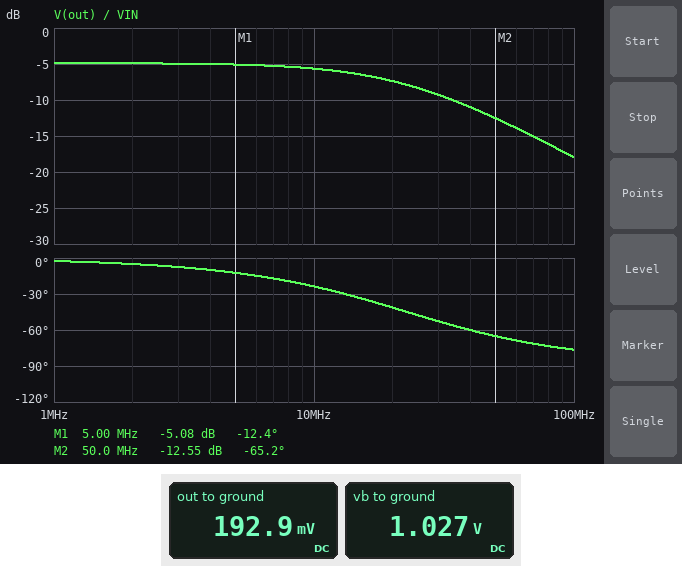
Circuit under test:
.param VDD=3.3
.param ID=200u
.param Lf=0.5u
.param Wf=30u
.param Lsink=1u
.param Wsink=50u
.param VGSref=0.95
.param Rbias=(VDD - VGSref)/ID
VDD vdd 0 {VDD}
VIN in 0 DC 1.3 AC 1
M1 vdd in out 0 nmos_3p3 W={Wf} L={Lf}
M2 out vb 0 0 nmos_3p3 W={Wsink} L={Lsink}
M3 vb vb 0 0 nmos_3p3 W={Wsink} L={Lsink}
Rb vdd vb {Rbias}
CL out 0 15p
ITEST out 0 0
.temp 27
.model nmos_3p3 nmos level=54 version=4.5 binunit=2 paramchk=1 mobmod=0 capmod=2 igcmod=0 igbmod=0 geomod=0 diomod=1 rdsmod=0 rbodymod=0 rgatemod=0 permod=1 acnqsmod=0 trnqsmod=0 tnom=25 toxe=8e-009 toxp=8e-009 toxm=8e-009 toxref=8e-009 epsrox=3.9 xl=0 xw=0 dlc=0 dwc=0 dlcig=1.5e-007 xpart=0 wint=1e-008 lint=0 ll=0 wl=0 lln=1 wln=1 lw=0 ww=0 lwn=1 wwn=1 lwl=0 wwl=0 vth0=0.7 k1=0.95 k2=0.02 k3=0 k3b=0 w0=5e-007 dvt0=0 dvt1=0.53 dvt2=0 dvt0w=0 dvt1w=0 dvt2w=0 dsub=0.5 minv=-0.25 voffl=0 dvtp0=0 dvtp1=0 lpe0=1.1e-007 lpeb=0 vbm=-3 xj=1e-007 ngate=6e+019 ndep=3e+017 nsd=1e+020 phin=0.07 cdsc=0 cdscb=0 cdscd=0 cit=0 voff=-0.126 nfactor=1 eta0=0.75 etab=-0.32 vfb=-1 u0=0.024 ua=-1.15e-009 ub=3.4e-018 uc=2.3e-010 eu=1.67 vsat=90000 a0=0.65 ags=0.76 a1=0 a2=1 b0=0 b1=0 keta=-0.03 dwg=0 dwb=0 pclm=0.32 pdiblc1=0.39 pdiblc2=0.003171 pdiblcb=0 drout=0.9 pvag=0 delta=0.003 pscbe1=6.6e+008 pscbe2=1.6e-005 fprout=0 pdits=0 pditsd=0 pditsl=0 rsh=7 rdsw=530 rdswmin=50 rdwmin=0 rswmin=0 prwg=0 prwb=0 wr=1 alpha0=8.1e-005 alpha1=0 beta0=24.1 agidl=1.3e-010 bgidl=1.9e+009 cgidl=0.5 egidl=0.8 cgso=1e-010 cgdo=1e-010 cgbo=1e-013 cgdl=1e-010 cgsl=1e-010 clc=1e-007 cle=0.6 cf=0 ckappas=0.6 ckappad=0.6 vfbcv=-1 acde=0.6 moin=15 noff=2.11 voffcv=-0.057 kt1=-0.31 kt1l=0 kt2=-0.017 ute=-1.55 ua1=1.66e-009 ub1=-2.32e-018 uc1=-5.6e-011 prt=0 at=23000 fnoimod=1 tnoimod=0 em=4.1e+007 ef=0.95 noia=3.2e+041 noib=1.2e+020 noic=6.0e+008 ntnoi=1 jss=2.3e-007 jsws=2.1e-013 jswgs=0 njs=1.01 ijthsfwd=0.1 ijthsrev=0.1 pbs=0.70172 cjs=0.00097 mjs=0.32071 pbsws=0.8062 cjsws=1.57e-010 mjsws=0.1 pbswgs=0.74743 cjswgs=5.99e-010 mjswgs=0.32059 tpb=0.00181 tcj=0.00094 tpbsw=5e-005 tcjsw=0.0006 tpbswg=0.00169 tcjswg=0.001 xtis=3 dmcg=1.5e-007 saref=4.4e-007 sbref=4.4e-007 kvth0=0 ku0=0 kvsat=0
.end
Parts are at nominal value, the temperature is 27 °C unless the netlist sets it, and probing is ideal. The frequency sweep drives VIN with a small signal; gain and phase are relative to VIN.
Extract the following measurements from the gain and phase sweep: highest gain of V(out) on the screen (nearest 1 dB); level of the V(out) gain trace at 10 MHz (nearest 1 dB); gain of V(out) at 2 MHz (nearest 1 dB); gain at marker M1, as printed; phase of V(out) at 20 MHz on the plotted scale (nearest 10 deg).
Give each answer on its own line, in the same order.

-5 dB
-6 dB
-5 dB
-5.08 dB
-40 deg
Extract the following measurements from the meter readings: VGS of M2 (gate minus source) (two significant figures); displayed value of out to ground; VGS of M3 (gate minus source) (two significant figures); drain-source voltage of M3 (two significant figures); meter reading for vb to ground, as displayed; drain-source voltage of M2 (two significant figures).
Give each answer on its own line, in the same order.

1.0 V
192.9 mV
1.0 V
1.0 V
1.027 V
190 mV
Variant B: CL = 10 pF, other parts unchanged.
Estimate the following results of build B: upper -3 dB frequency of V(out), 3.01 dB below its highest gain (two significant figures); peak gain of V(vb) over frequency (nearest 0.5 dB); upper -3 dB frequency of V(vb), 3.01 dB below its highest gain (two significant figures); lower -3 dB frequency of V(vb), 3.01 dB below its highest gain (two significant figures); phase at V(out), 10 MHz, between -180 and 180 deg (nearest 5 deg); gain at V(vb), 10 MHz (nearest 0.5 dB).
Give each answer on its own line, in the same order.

34 MHz
-51.5 dB
690 MHz
31 MHz
-15 deg
-62.0 dB
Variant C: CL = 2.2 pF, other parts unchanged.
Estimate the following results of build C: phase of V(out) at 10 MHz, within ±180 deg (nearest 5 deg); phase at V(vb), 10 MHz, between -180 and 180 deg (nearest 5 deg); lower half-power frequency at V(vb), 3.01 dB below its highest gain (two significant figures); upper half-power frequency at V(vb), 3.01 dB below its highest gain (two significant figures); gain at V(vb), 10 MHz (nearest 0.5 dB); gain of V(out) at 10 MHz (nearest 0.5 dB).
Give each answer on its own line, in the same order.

-5 deg
85 deg
100 MHz
880 MHz
-61.5 dB
-5.0 dB
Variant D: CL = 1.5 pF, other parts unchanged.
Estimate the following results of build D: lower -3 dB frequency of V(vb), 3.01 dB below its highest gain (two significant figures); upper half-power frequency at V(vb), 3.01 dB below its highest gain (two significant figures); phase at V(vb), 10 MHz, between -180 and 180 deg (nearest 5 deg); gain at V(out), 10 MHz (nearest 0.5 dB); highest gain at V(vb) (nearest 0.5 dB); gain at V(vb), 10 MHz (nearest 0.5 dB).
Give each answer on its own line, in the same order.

130 MHz
980 MHz
85 deg
-5.0 dB
-38.0 dB
-61.5 dB
